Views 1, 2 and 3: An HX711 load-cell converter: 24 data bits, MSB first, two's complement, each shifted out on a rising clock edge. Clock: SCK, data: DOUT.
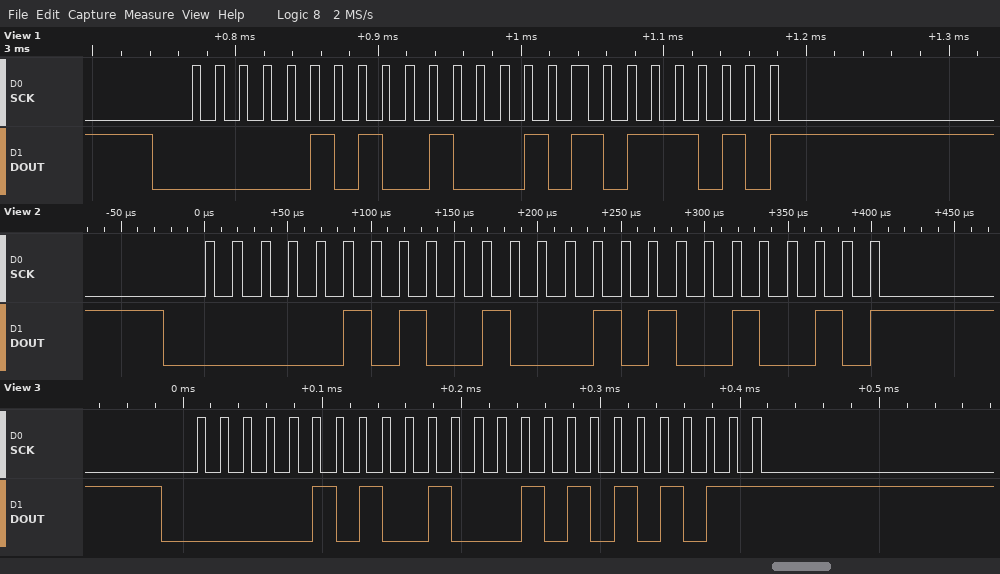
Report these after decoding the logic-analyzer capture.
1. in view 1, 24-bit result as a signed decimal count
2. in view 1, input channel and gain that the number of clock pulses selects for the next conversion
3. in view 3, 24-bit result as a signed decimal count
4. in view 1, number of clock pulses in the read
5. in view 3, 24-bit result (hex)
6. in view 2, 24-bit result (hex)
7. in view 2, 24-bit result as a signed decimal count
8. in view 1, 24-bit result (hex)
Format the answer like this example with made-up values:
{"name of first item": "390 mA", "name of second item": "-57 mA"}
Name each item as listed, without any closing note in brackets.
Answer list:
{"in view 1, 24-bit result as a signed decimal count": "336570", "in view 1, input channel and gain that the number of clock pulses selects for the next conversion": "channel A, gain 128", "in view 3, 24-bit result as a signed decimal count": "336555", "in view 1, number of clock pulses in the read": "25", "in view 3, 24-bit result": "0x0522AB", "in view 2, 24-bit result": "0x052292", "in view 2, 24-bit result as a signed decimal count": "336530", "in view 1, 24-bit result": "0x0522BA"}
